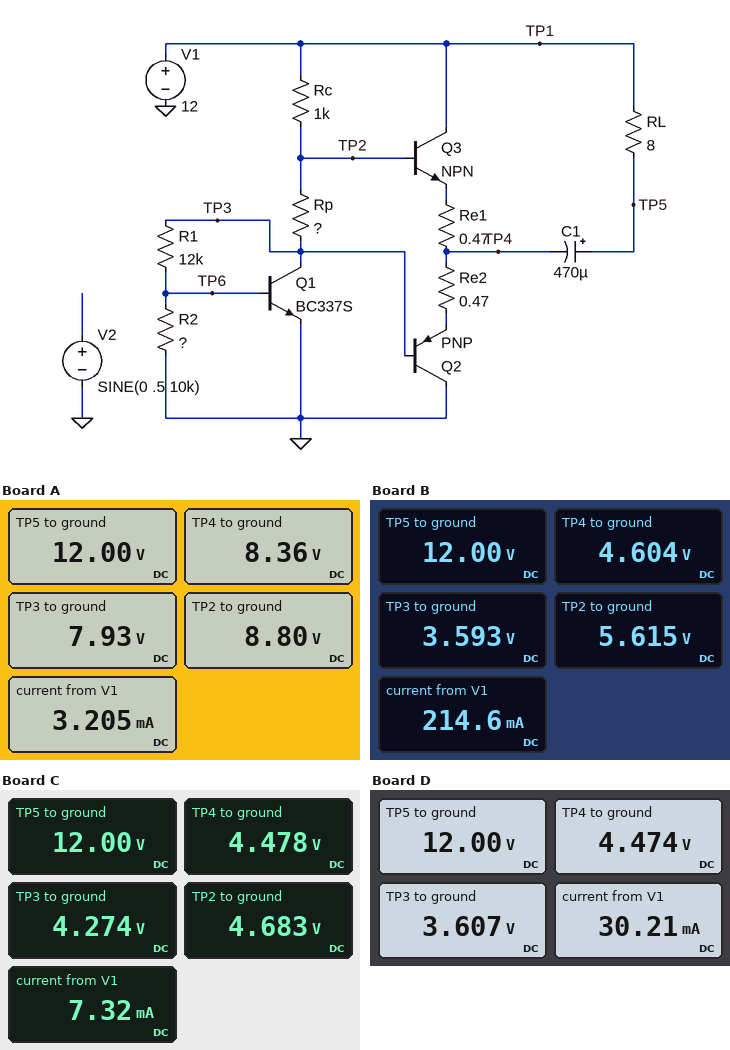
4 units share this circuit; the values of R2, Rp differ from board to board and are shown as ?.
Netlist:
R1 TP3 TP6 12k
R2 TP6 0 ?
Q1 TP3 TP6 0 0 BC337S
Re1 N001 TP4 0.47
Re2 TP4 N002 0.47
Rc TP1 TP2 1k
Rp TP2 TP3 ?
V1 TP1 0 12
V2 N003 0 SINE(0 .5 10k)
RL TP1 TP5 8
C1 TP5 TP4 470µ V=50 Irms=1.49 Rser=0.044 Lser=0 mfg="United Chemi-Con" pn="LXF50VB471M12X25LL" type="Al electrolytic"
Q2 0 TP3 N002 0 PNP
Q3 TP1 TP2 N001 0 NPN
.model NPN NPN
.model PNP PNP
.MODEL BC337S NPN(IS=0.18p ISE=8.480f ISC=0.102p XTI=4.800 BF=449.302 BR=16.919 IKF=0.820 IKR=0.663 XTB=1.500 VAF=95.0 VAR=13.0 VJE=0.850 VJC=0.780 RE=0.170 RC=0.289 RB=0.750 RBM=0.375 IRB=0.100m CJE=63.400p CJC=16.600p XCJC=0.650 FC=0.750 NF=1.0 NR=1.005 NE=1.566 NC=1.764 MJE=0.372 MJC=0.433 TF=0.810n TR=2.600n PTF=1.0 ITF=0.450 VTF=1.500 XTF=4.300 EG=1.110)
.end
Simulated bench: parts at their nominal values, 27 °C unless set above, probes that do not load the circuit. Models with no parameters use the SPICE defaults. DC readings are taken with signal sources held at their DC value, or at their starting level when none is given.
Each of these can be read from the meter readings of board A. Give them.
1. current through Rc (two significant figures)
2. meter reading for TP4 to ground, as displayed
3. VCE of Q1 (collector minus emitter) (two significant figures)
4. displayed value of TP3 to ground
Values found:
3.2 mA
8.36 V
7.9 V
7.93 V
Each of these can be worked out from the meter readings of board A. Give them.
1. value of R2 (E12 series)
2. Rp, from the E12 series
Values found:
1 kΩ
270 Ω
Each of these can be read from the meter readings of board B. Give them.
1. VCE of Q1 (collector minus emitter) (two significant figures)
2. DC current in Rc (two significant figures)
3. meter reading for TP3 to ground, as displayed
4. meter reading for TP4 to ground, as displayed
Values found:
3.6 V
6.4 mA
3.593 V
4.604 V
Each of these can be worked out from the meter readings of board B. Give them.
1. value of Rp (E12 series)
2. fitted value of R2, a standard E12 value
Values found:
470 Ω
2.7 kΩ
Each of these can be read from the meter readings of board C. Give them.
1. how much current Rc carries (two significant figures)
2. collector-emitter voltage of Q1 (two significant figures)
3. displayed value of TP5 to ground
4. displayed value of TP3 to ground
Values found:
7.3 mA
4.3 V
12.00 V
4.274 V
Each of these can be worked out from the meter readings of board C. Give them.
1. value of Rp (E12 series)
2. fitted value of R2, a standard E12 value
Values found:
56 Ω
2.2 kΩ
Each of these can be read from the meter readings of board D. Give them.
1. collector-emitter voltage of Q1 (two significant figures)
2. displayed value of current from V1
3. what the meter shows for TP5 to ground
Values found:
3.6 V
30.21 mA
12.00 V
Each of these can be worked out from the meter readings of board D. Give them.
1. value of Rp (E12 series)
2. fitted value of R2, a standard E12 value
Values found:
270 Ω
2.7 kΩ
